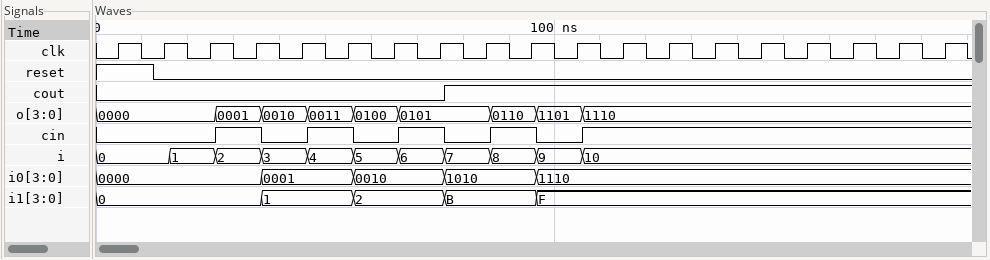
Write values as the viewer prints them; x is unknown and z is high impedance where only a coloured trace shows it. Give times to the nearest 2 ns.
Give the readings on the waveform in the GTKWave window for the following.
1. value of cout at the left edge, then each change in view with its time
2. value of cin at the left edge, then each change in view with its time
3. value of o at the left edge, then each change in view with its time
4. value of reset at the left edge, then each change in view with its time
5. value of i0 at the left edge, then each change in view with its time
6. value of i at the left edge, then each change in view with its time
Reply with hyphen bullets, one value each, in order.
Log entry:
- 0, 1 at 76 ns
- 0, 1 at 26 ns, 0 at 36 ns, 1 at 46 ns, 0 at 56 ns, 1 at 66 ns, 0 at 76 ns, 1 at 86 ns, 0 at 96 ns, 1 at 106 ns
- 0000, 0001 at 26 ns, 0010 at 36 ns, 0011 at 46 ns, 0100 at 56 ns, 0101 at 66 ns, 0110 at 86 ns, 1101 at 96 ns, 1110 at 106 ns
- 1, 0 at 12 ns
- 0000, 0001 at 36 ns, 0010 at 56 ns, 1010 at 76 ns, 1110 at 96 ns
- 0, 1 at 16 ns, 2 at 26 ns, 3 at 36 ns, 4 at 46 ns, 5 at 56 ns, 6 at 66 ns, 7 at 76 ns, 8 at 86 ns, 9 at 96 ns, 10 at 106 ns
